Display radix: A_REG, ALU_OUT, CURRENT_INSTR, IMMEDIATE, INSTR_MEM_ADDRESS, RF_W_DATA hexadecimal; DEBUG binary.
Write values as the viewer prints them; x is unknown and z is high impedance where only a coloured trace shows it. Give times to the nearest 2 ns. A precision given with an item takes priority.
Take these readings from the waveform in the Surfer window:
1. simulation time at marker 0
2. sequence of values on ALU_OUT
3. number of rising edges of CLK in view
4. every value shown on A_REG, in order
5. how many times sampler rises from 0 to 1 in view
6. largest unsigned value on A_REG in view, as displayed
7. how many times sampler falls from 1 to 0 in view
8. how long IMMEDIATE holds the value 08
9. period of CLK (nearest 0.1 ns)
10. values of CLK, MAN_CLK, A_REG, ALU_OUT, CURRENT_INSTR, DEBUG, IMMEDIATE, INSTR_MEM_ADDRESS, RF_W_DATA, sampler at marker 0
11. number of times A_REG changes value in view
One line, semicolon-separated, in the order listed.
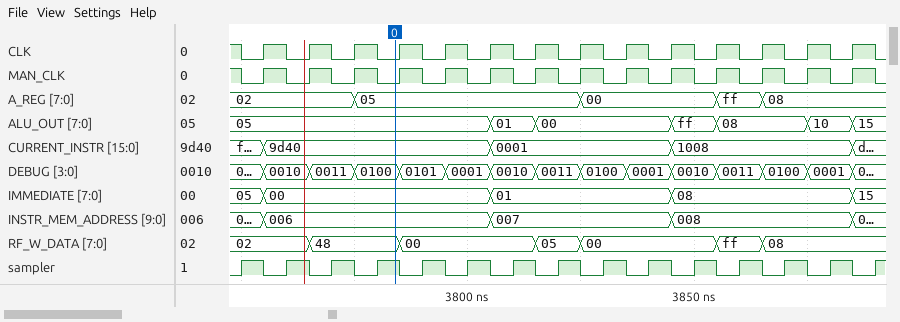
3784 ns; 05, 01, 00, ff, 08, 10, 15; 14; 02, 05, 00, ff, 08; 15; ff; 14; 40 ns; 10 ns; CLK=0, MAN_CLK=0, A_REG=05, ALU_OUT=05, CURRENT_INSTR=9d40, DEBUG=0100, IMMEDIATE=00, INSTR_MEM_ADDRESS=006, RF_W_DATA=48, sampler=1; 4
